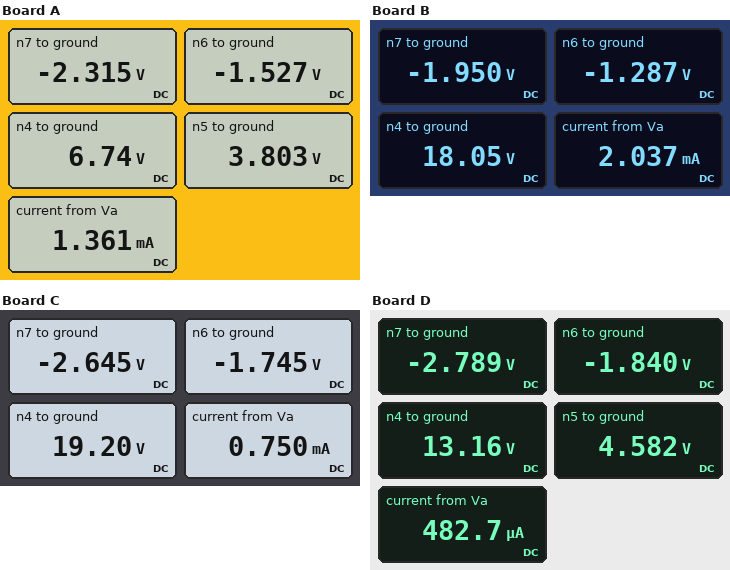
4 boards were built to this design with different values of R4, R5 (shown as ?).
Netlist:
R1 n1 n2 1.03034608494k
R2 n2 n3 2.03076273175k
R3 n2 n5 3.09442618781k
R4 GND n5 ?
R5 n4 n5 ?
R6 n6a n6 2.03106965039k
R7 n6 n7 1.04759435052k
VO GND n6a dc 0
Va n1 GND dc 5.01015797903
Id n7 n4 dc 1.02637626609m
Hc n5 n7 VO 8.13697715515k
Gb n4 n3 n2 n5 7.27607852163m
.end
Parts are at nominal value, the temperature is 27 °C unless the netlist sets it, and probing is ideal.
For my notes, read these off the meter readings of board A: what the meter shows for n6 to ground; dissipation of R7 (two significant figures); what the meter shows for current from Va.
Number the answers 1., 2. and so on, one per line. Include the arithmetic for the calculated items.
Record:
1. -1.527 V
2. (-1.527 V - (-2.315 V))^2 / 1.048 kΩ = 590 µW
3. 1.361 mA
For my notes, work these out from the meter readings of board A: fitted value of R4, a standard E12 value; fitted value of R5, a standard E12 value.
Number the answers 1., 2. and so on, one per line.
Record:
1. 1.8 kΩ
2. 1.2 kΩ
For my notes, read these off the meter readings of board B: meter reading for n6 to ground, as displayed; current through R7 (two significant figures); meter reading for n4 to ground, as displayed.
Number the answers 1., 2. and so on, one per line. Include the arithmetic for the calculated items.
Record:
1. -1.287 V
2. (-1.287 V - (-1.95 V)) / 1.048 kΩ = 630 µA
3. 18.05 V
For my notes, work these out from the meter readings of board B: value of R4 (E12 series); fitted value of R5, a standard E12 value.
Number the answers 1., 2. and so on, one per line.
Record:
1. 1.2 kΩ
2. 4.7 kΩ
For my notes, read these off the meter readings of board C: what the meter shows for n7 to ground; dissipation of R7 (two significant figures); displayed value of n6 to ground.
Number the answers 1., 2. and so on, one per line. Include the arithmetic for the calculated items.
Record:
1. -2.645 V
2. (-1.745 V - (-2.645 V))^2 / 1.048 kΩ = 770 µW
3. -1.745 V
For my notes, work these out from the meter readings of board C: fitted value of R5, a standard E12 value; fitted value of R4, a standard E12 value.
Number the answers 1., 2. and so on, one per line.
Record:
1. 8.2 kΩ
2. 2.7 kΩ
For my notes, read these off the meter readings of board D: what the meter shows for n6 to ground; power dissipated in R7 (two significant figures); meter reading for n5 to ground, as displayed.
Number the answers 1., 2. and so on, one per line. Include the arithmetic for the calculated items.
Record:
1. -1.840 V
2. (-1.84 V - (-2.789 V))^2 / 1.048 kΩ = 860 µW
3. 4.582 V
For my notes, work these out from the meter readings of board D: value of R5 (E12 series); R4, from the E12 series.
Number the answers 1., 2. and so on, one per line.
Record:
1. 5.6 kΩ
2. 3.3 kΩ
